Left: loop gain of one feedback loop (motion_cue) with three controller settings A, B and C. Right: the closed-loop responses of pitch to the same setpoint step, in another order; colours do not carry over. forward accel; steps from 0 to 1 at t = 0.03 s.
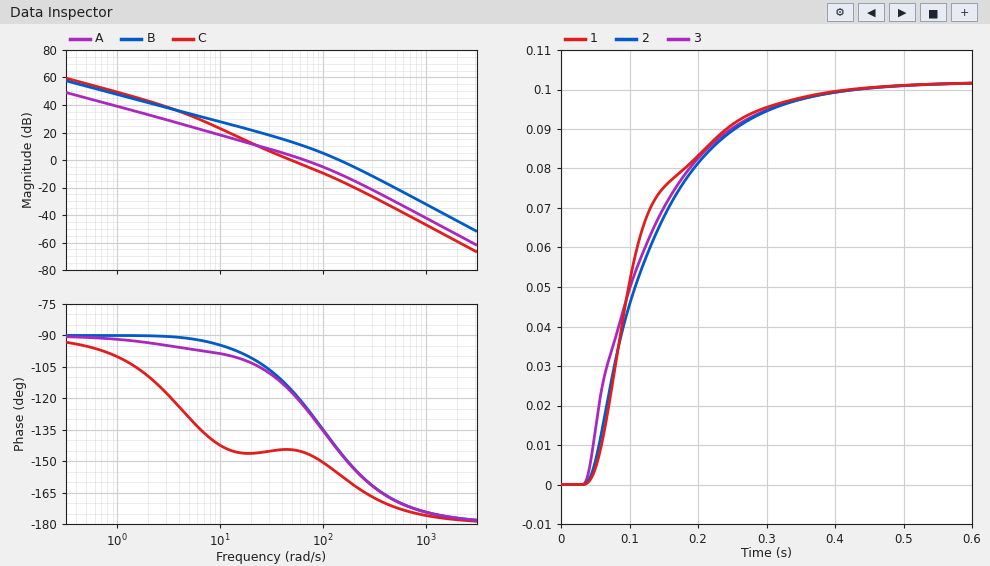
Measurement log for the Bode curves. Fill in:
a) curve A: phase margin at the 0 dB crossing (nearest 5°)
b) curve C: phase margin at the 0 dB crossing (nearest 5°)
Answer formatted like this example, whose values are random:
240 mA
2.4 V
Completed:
55°
35°
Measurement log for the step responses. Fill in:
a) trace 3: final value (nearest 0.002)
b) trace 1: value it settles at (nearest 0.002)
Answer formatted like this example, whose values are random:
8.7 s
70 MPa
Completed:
0.102
0.102
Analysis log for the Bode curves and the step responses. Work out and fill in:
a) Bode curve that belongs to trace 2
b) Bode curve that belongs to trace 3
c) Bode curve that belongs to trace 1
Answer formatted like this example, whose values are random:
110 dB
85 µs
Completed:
A
B
C
